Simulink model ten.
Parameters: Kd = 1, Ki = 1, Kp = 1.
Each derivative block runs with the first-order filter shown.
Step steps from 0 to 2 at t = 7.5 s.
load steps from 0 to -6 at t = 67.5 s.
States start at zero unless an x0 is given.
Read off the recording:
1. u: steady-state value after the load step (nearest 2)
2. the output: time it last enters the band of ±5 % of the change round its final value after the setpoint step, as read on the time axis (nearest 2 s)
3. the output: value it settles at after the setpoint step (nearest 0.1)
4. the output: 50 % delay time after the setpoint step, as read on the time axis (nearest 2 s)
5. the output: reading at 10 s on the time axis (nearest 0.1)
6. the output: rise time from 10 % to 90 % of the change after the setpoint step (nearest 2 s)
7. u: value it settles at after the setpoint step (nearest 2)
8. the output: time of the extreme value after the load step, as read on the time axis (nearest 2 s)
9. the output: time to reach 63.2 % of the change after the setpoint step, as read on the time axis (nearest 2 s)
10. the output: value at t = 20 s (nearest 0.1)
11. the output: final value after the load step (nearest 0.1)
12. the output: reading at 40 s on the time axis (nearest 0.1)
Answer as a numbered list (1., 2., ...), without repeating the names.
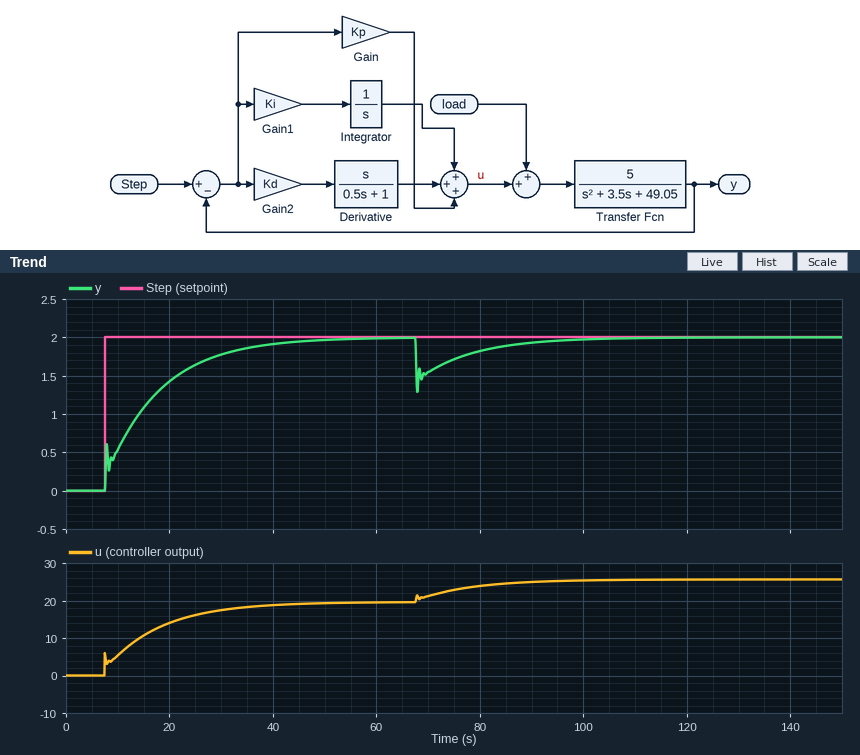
1. 26
2. 38 s
3. 2.0
4. 14 s
5. 0.5
6. 24 s
7. 20
8. 68 s
9. 18 s
10. 1.4
11. 2.0
12. 1.9
